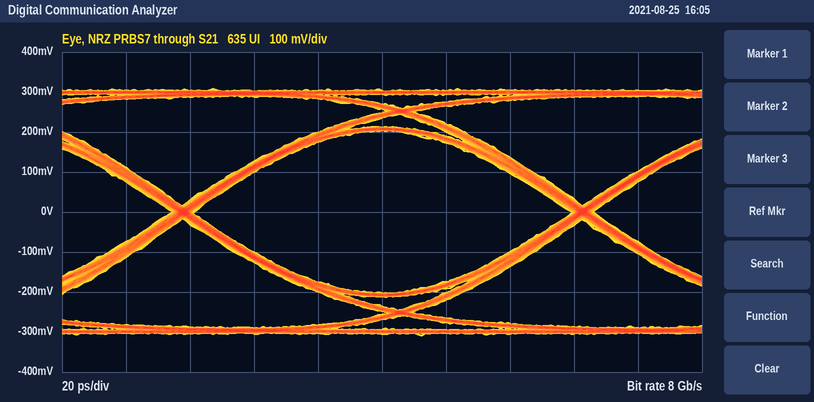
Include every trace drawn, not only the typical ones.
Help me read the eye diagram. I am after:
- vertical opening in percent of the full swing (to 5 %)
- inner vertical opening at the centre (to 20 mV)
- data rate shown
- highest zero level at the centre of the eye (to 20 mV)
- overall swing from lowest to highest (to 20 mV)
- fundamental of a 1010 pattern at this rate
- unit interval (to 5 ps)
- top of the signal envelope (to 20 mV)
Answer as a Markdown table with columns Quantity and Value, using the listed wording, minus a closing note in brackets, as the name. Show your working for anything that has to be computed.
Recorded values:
| Quantity | Value |
|---|---|
| vertical opening in percent of the full swing | 400 mV / 620 mV ≈ 65 % |
| inner vertical opening at the centre | 400 mV |
| data rate shown | 8 Gb/s |
| highest zero level at the centre of the eye | -200 mV |
| overall swing from lowest to highest | 620 mV |
| fundamental of a 1010 pattern at this rate | 4 GHz |
| unit interval | 125 ps |
| top of the signal envelope | 300 mV |
